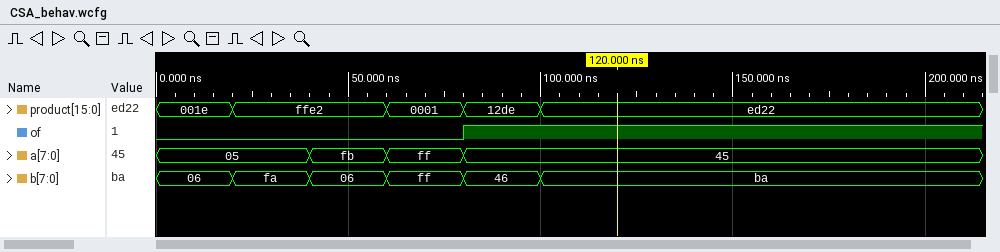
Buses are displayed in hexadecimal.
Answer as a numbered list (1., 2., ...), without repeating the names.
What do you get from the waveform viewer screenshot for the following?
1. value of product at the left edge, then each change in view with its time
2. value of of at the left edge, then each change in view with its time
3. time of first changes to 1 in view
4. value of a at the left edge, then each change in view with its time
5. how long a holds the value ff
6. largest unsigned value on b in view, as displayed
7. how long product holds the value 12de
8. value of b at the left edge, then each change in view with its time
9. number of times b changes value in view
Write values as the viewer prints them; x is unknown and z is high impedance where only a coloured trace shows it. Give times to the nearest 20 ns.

1. 001e, ffe2 at 20 ns, 0001 at 60 ns, 12de at 80 ns, ed22 at 100 ns
2. 0, 1 at 80 ns
3. 80 ns
4. 05, fb at 40 ns, ff at 60 ns, 45 at 80 ns
5. 20 ns
6. ff
7. 20 ns
8. 06, fa at 20 ns, 06 at 40 ns, ff at 60 ns, 46 at 80 ns, ba at 100 ns
9. 5
